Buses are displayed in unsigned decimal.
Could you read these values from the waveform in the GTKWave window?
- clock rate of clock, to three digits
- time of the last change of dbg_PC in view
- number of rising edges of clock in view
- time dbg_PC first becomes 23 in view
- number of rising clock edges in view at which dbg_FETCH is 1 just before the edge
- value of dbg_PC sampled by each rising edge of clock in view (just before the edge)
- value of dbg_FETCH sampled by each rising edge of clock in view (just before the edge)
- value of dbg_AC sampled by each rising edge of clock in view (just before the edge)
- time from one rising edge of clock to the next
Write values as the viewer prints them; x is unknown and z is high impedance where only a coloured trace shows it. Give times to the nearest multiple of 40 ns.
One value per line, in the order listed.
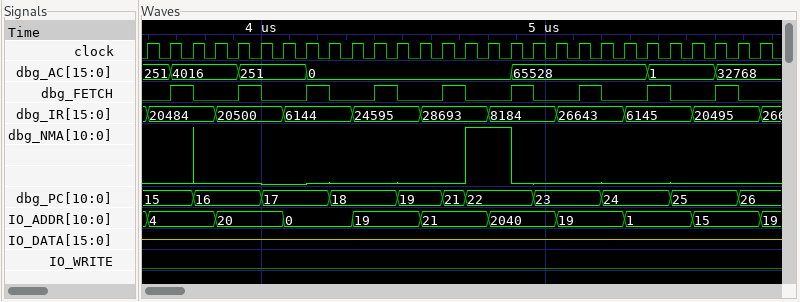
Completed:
12.5 MHz
5680 ns
28
4960 ns
9
15, 15, 15, 16, 16, 16, 17, 17, 17, 18, 18, 18, 19, 19, 21, 22, 22, 22, 23, 23, 23, 24, 24, 24, 25, 25, 25, 26
0 0 1 0 0 1 0 0 1 0 0 1 0 0 1 0 0 1 0 0 1 0 0 1 0 0 1 0
251, 251, 4016, 4016, 4016, 251, 251, 251, 0, 0, 0, 0, 0, 0, 0, 0, 0, 65528, 65528, 65528, 65528, 65528, 65528, 1, 1, 1, 32768, 32768
80 ns
